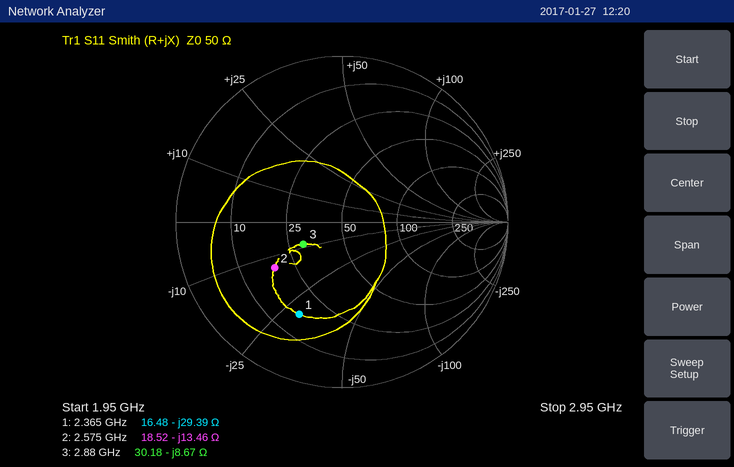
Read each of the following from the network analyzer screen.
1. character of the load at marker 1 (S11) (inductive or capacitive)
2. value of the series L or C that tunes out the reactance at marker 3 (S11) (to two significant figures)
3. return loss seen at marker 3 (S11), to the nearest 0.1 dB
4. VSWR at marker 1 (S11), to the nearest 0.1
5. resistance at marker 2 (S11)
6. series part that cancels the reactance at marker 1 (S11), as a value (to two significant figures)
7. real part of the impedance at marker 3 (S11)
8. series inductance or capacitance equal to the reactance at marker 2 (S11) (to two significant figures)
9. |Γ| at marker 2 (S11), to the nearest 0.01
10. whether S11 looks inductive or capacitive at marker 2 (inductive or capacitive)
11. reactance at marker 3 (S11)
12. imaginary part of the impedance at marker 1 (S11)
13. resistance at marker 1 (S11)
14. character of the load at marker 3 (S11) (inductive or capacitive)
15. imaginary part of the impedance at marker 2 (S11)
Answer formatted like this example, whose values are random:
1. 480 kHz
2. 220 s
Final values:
1. capacitive
2. 480 pH
3. 11.4 dB
4. 4.2
5. 18.52 Ω
6. 2.0 nH
7. 30.18 Ω
8. 4.6 pF
9. 0.49
10. capacitive
11. -8.67 Ω
12. -29.39 Ω
13. 16.48 Ω
14. capacitive
15. -13.46 Ω
